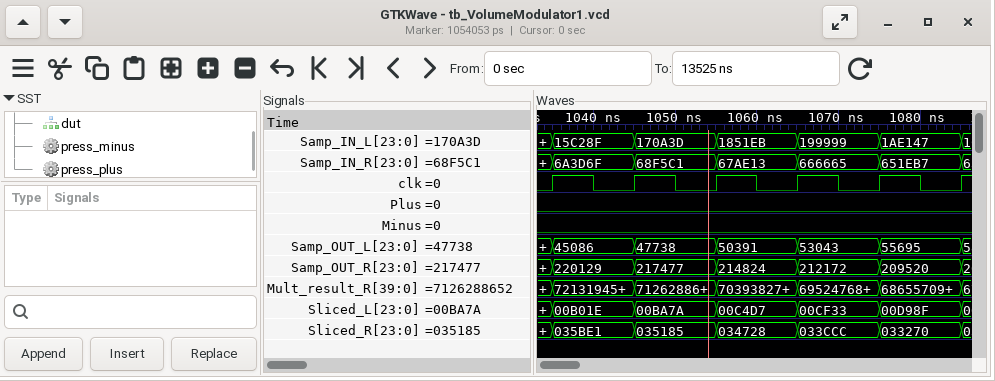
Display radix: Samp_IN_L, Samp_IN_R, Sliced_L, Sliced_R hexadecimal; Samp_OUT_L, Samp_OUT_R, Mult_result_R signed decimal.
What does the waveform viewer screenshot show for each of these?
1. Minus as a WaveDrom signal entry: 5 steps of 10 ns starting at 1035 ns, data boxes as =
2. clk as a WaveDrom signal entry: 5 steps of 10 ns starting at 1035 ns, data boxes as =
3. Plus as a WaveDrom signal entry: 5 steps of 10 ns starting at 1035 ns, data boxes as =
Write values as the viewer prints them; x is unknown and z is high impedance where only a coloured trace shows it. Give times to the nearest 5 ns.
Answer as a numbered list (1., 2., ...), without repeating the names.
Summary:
1. {name: 'Minus', wave: '0....'}
2. {name: 'clk', wave: 'p....'}
3. {name: 'Plus', wave: '0....'}
